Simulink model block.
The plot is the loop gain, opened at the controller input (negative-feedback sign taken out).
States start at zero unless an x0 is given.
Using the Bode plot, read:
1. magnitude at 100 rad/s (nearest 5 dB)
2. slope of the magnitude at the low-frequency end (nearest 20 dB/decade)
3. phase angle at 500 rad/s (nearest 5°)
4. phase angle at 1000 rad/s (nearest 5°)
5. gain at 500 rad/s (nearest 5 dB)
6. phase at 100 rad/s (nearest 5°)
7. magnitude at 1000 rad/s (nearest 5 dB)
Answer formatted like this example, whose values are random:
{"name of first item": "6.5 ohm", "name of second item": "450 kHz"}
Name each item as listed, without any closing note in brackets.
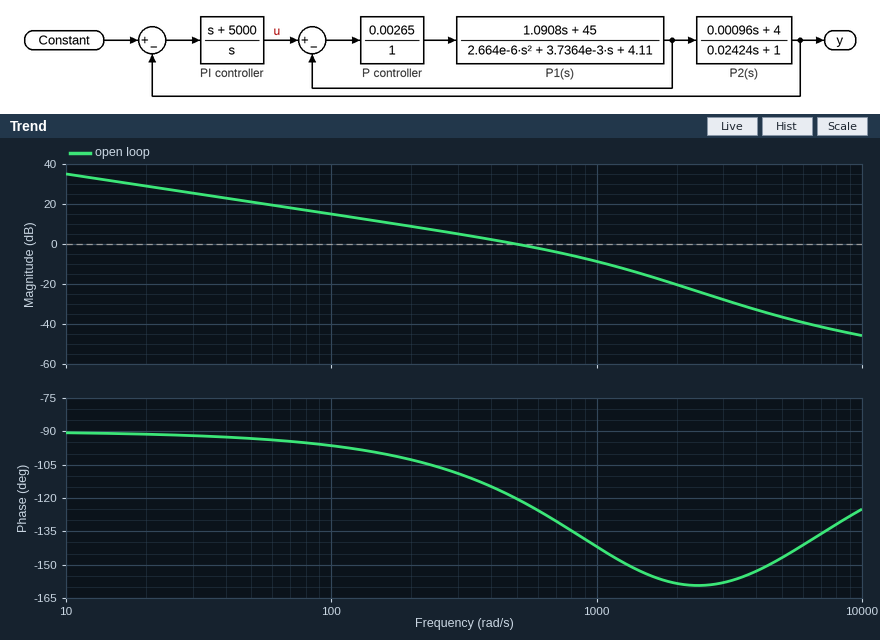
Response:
{"magnitude at 100 rad/s": "15 dB", "slope of the magnitude at the low-frequency end": "-20 dB/decade", "phase angle at 500 rad/s": "-120°", "phase angle at 1000 rad/s": "-140°", "gain at 500 rad/s": "0 dB", "phase at 100 rad/s": "-95°", "magnitude at 1000 rad/s": "-10 dB"}
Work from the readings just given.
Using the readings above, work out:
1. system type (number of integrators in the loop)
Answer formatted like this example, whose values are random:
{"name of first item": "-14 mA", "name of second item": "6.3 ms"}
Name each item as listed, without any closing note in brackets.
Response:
{"system type": "1"}
